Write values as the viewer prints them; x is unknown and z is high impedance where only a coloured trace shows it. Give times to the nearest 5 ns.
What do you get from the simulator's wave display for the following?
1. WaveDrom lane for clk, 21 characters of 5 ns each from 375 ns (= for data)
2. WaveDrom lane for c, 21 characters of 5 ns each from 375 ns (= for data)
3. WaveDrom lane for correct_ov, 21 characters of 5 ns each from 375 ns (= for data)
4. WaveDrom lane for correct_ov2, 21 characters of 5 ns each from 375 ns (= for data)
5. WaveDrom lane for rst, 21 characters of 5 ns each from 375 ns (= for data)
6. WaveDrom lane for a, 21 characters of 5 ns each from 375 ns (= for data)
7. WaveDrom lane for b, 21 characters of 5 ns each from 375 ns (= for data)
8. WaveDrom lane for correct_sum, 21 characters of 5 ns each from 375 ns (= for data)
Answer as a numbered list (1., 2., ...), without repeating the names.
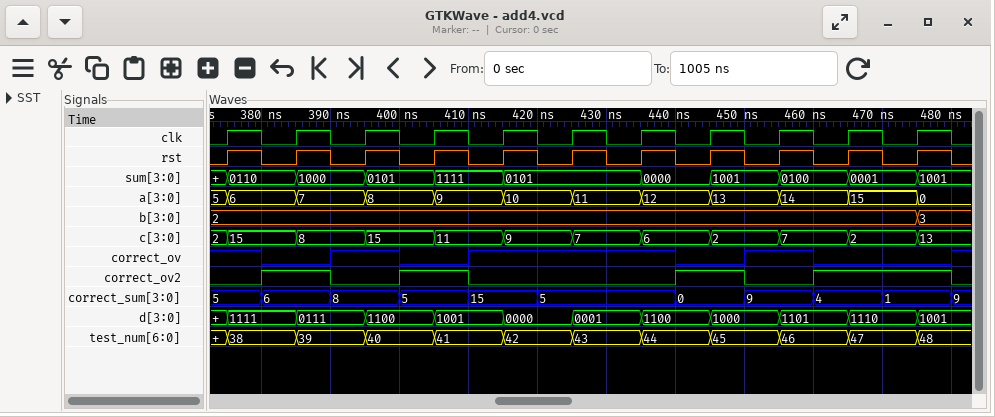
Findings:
1. {name: 'clk', wave: '101010101010101010101'}
2. {name: 'c', wave: '=.=.=.=.=.=.=.=.=.=.=', data: '15 8 15 11 9 7 6 2 7 2 13'}
3. {name: 'correct_ov', wave: '10.1.0.1.....0.1.0...'}
4. {name: 'correct_ov2', wave: '01.0.1.0.....1.0.1...'}
5. {name: 'rst', wave: '101010101010101010101'}
6. {name: 'a', wave: '=.=.=.=.=.=.=.=.=.=.=', data: '6 7 8 9 10 11 12 13 14 15 0'}
7. {name: 'b', wave: '=...................=', data: '2 3'}
8. {name: 'correct_sum', wave: '==.=.=.=.=...=.=.=.=.', data: '5 6 8 5 15 5 0 9 4 1'}
